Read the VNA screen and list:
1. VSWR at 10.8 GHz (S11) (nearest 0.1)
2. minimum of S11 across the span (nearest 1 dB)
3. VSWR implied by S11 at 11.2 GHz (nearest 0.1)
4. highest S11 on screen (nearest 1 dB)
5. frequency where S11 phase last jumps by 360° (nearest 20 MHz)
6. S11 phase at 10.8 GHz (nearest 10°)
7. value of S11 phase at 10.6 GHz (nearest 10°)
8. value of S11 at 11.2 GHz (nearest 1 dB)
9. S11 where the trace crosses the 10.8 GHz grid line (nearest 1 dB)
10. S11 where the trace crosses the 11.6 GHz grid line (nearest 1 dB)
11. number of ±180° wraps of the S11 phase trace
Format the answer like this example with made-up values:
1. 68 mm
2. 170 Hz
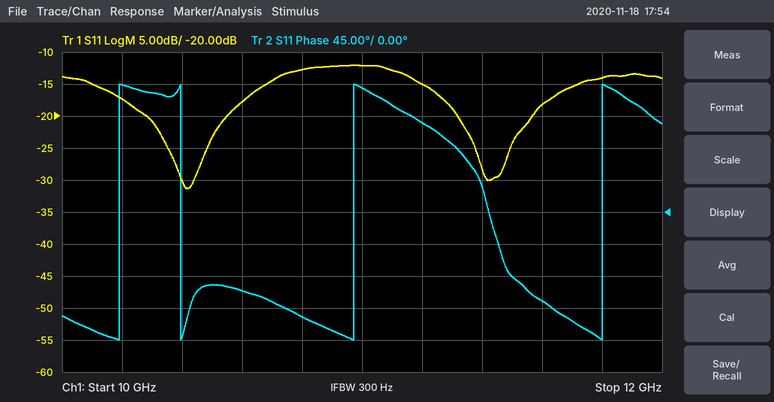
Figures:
1. 1.6
2. -31 dB
3. 1.4
4. -12 dB
5. 11.80 GHz
6. -150°
7. -110°
8. -15 dB
9. -13 dB
10. -18 dB
11. 4
